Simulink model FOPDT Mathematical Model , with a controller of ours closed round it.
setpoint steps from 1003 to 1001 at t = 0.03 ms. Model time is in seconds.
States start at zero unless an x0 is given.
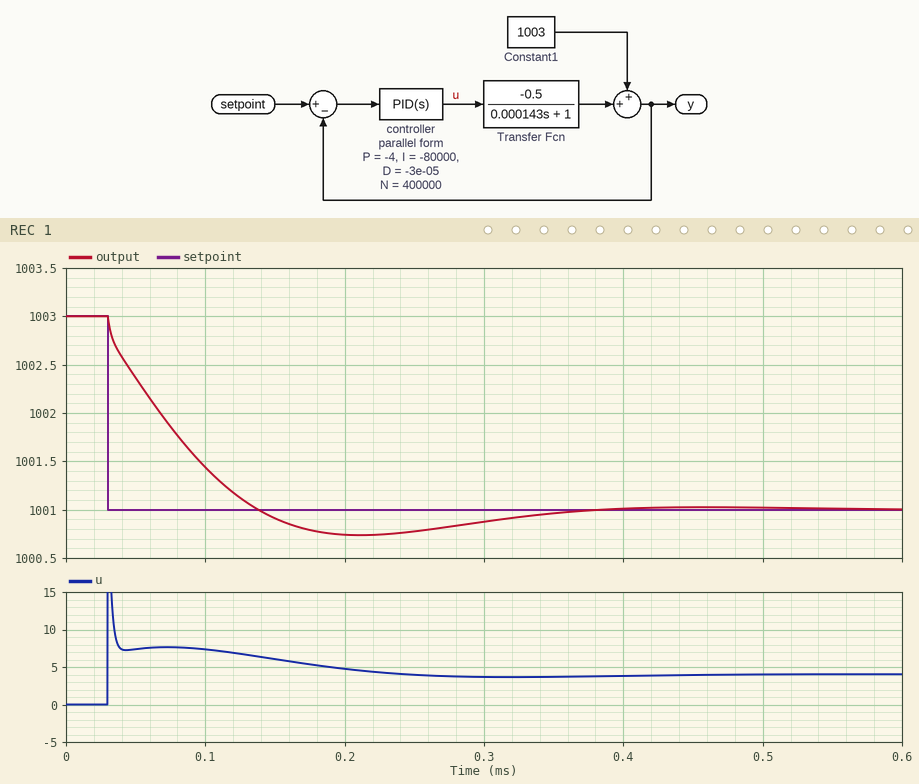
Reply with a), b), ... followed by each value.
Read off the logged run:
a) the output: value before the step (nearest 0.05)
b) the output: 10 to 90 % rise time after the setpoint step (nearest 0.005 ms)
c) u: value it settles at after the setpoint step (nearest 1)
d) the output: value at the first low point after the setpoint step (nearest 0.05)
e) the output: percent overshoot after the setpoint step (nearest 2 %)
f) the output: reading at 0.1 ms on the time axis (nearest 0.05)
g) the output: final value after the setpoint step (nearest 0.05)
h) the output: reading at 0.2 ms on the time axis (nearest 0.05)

a) 1003.00
b) 0.085 ms
c) 4
d) 1000.75
e) 14 %
f) 1001.45
g) 1001.00
h) 1000.75
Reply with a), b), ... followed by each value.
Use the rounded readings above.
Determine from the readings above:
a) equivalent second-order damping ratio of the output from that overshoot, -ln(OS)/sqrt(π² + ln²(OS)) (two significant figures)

a) 0.53
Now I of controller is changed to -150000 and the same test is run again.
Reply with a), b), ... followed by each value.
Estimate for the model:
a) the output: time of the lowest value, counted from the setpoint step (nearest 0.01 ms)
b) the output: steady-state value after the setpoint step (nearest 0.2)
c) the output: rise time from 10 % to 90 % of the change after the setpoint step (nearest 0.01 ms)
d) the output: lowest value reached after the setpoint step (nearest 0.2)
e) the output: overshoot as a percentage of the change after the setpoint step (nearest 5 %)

a) 0.13 ms
b) 1001.0
c) 0.06 ms
d) 1000.6
e) 25 %
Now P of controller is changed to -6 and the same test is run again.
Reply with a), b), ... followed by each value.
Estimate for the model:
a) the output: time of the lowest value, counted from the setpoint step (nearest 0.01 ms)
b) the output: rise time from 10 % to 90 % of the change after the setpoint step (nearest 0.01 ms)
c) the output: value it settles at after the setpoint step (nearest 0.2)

a) 0.18 ms
b) 0.08 ms
c) 1001.0
